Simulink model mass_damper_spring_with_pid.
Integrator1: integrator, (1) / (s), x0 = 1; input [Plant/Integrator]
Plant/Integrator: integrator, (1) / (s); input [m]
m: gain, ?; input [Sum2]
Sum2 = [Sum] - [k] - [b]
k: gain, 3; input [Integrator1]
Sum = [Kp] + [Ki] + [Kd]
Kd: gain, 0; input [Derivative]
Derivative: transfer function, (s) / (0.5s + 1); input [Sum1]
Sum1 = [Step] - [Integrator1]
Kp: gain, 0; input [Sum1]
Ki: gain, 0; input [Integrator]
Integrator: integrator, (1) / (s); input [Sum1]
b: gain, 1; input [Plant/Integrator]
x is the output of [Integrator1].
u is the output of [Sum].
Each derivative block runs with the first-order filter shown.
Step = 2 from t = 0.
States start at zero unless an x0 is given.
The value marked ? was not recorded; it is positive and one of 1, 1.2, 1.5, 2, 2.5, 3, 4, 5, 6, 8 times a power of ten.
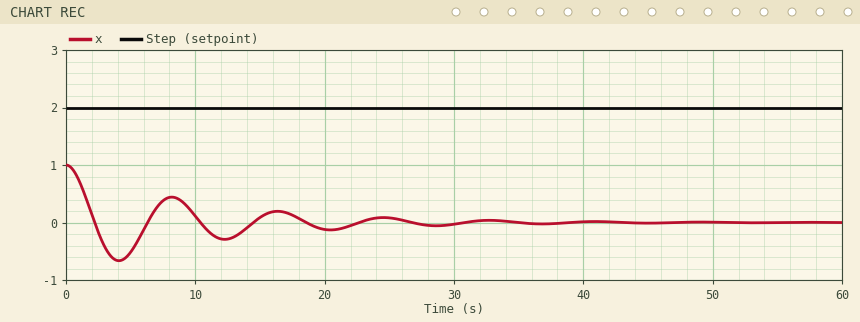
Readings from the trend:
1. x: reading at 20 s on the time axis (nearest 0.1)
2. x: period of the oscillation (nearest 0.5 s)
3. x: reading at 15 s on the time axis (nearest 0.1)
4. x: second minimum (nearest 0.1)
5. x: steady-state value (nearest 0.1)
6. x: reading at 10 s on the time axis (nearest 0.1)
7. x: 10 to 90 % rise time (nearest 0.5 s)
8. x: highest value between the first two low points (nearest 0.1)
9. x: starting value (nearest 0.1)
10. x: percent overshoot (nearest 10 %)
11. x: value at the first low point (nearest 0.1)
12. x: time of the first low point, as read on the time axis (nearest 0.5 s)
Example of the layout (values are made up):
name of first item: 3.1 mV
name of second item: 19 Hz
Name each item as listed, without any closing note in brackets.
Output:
x: reading at 20 s on the time axis: -0.1
x: period of the oscillation: 8.0 s
x: reading at 15 s on the time axis: 0.1
x: second minimum: -0.3
x: steady-state value: 0.0
x: reading at 10 s on the time axis: 0.1
x: 10 to 90 % rise time: 1.5 s
x: highest value between the first two low points: 0.4
x: starting value: 1.0
x: percent overshoot: 70 %
x: value at the first low point: -0.7
x: time of the first low point, as read on the time axis: 4.0 s
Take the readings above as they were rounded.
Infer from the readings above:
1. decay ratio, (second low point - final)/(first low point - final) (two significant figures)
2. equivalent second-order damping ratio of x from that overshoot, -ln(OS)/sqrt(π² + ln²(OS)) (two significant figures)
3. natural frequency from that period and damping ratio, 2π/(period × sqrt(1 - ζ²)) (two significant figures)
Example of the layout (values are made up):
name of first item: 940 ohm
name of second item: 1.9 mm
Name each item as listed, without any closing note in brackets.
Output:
decay ratio, (second low point - final)/(first low point - final): 0.43
equivalent second-order damping ratio of x from that overshoot, -ln(OS)/sqrt(π² + ln²(OS)): 0.11
natural frequency from that period and damping ratio, 2π/(period × sqrt(1 - ζ²)): 0.79 rad/s
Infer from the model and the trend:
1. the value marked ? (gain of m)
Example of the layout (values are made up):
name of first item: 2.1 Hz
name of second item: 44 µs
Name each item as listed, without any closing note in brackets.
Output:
the value marked ?: 0.2
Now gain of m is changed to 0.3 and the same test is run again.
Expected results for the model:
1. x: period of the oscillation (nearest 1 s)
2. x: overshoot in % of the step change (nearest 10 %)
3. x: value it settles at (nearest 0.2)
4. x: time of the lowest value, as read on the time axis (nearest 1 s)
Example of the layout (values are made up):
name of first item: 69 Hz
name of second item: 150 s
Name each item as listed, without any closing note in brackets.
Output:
x: period of the oscillation: 7 s
x: overshoot in % of the step change: 60 %
x: value it settles at: 0.0
x: time of the lowest value, as read on the time axis: 3 s
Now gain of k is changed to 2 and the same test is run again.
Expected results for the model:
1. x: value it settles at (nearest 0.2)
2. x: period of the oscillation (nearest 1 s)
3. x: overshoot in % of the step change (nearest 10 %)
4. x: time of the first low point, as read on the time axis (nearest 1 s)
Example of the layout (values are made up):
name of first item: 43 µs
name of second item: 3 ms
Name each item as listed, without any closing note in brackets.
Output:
x: value it settles at: 0.0
x: period of the oscillation: 10 s
x: overshoot in % of the step change: 60 %
x: time of the first low point, as read on the time axis: 5 s
